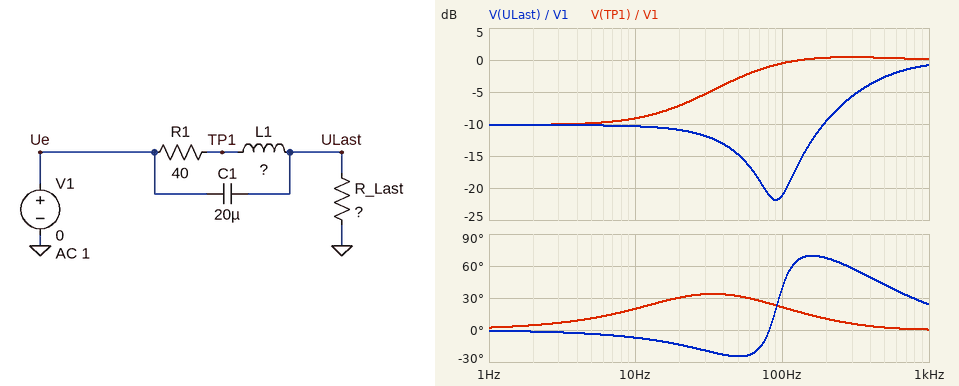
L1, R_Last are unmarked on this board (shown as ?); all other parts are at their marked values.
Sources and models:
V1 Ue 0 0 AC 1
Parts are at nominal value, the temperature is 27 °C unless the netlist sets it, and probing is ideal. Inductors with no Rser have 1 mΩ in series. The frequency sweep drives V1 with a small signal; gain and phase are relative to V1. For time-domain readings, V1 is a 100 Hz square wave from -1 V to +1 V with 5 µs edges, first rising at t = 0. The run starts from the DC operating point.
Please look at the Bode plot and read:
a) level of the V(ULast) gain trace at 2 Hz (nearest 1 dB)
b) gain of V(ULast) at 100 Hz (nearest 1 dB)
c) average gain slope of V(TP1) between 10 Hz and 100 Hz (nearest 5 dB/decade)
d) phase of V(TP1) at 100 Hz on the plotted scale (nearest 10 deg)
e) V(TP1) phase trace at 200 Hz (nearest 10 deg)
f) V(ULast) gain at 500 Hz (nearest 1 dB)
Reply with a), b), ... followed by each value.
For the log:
a) -10 dB
b) -21 dB
c) 10 dB/decade
d) 20 deg
e) 10 deg
f) -3 dB
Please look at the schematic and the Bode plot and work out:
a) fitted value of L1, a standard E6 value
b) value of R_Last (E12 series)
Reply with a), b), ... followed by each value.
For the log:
a) 150 mH
b) 18 Ω
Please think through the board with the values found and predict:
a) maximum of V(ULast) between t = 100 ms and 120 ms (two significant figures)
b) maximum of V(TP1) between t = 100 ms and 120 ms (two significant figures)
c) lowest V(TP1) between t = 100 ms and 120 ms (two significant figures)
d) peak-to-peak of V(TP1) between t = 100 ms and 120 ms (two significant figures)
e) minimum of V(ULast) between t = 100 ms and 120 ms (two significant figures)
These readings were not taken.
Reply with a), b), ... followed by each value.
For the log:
a) 1.8 V
b) 1.5 V
c) -1.5 V
d) 3.0 V
e) -1.8 V
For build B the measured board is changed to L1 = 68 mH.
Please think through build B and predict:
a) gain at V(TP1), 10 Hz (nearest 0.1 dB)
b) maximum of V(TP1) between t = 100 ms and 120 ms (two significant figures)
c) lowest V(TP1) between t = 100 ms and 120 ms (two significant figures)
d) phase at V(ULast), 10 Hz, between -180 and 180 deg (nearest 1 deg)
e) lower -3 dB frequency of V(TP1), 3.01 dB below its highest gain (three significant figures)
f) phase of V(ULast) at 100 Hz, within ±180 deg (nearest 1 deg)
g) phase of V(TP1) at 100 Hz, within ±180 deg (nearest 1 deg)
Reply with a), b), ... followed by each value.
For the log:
a) -9.9 dB
b) 1.7 V
c) -1.7 V
d) -2 deg
e) 107 Hz
f) 0 deg
g) 34 deg
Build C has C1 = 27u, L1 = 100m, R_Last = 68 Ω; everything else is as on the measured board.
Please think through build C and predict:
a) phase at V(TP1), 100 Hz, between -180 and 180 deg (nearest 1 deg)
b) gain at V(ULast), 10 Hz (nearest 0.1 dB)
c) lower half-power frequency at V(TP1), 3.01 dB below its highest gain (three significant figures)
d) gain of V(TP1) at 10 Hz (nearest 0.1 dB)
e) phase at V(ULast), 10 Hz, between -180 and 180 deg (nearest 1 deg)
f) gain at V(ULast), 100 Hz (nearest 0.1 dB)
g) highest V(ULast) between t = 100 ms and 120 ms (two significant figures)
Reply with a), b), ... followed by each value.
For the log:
a) 20 deg
b) -4.1 dB
c) 68.5 Hz
d) -4.0 dB
e) -2 deg
f) -7.9 dB
g) 1.5 V
